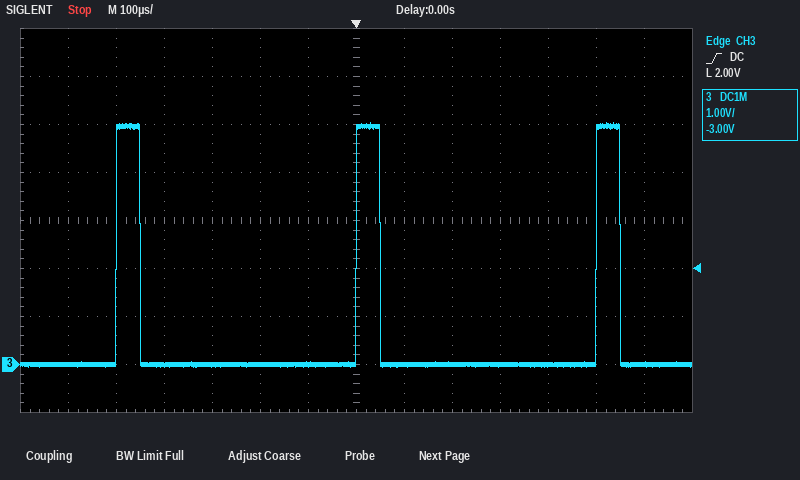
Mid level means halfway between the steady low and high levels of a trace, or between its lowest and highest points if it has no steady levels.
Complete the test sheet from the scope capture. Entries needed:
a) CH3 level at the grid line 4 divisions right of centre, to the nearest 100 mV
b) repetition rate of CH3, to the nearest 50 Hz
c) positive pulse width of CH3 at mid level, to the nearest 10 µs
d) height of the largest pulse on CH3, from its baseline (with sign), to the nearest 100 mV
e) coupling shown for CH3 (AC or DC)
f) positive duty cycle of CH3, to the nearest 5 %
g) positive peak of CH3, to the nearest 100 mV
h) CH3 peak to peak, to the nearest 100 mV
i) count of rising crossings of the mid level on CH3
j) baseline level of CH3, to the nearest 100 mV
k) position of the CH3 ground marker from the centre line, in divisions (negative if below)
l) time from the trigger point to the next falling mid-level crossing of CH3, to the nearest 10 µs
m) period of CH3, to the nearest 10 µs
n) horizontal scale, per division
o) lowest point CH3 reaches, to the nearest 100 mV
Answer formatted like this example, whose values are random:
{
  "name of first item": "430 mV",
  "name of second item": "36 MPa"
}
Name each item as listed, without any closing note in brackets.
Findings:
{
  "CH3 level at the grid line 4 divisions right of centre, to the nearest 100 mV": "0.0 V",
  "repetition rate of CH3, to the nearest 50 Hz": "2.00 kHz",
  "positive pulse width of CH3 at mid level, to the nearest 10 µs": "50 µs",
  "height of the largest pulse on CH3, from its baseline (with sign), to the nearest 100 mV": "+5.0 V",
  "coupling shown for CH3": "DC",
  "positive duty cycle of CH3, to the nearest 5 %": "10 %",
  "positive peak of CH3, to the nearest 100 mV": "5.0 V",
  "CH3 peak to peak, to the nearest 100 mV": "5.1 V",
  "count of rising crossings of the mid level on CH3": "3",
  "baseline level of CH3, to the nearest 100 mV": "0.0 V",
  "position of the CH3 ground marker from the centre line, in divisions": "-3.0 div",
  "time from the trigger point to the next falling mid-level crossing of CH3, to the nearest 10 µs": "50 µs",
  "period of CH3, to the nearest 10 µs": "500 µs",
  "horizontal scale, per division": "100 µs",
  "lowest point CH3 reaches, to the nearest 100 mV": "-100 mV"
}
